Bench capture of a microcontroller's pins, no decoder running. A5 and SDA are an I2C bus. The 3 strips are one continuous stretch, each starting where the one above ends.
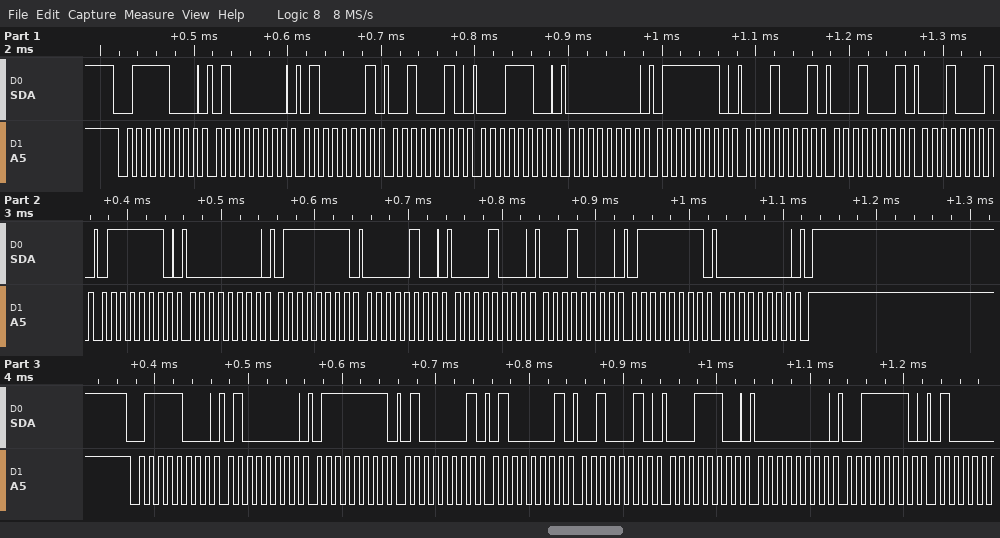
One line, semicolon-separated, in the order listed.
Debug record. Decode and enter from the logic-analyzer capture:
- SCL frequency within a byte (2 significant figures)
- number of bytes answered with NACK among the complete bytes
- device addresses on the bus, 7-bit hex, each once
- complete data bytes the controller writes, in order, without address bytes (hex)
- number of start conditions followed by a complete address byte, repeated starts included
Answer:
100 kHz; 0; 0x3C; 40 41 22 1C 00 7E 11 11 11 7E 00 7F 04 08 10 7F 00 40 7F 41 41 22 1C 00 3E; 2
